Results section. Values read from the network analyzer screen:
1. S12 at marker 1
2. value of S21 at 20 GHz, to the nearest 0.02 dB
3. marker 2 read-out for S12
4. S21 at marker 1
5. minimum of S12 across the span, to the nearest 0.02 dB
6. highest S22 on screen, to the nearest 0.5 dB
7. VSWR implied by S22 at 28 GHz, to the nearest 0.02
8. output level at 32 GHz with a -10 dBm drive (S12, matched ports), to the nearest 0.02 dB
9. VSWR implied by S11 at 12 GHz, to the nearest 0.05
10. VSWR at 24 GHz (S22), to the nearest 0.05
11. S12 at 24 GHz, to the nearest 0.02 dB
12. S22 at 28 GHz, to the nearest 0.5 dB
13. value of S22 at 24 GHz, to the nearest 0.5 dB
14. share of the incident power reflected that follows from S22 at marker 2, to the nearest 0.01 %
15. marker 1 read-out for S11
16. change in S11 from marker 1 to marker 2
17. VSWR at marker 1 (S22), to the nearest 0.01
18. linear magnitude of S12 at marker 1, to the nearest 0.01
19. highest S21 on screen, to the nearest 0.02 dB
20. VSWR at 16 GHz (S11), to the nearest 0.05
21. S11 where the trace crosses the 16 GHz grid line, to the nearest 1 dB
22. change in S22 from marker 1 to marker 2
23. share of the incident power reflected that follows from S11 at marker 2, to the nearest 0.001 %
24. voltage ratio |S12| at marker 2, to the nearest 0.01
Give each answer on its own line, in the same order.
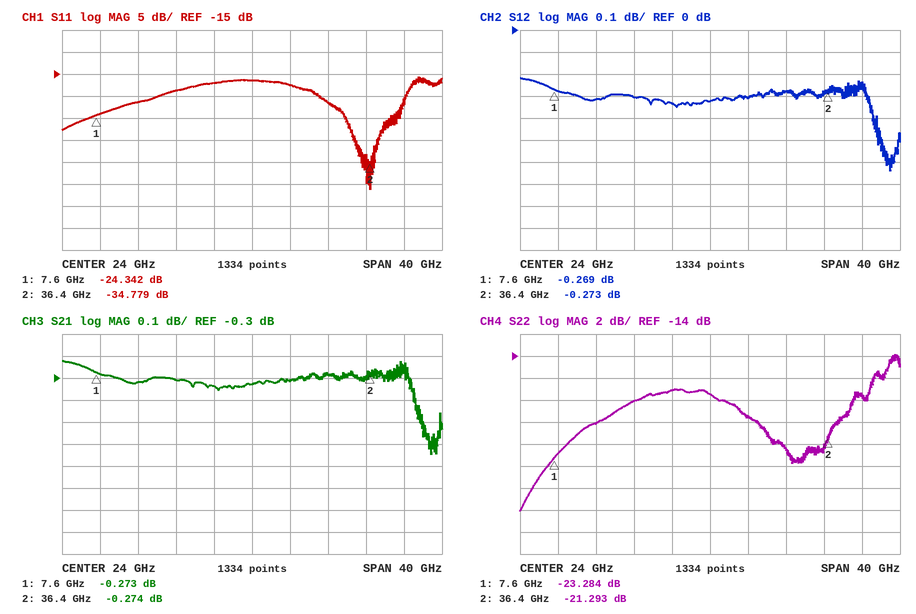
-0.269 dB
-0.34 dB
-0.273 dB
-0.273 dB
-0.64 dB
-14.0 dB
1.24
-10.28 dBm
1.20
1.30
-0.32 dB
-19.5 dB
-17.5 dB
0.74 %
-24.342 dB
-10.437 dB
1.15
0.97
-0.22 dB
1.25
-19 dB
1.991 dB
0.033 %
0.97
